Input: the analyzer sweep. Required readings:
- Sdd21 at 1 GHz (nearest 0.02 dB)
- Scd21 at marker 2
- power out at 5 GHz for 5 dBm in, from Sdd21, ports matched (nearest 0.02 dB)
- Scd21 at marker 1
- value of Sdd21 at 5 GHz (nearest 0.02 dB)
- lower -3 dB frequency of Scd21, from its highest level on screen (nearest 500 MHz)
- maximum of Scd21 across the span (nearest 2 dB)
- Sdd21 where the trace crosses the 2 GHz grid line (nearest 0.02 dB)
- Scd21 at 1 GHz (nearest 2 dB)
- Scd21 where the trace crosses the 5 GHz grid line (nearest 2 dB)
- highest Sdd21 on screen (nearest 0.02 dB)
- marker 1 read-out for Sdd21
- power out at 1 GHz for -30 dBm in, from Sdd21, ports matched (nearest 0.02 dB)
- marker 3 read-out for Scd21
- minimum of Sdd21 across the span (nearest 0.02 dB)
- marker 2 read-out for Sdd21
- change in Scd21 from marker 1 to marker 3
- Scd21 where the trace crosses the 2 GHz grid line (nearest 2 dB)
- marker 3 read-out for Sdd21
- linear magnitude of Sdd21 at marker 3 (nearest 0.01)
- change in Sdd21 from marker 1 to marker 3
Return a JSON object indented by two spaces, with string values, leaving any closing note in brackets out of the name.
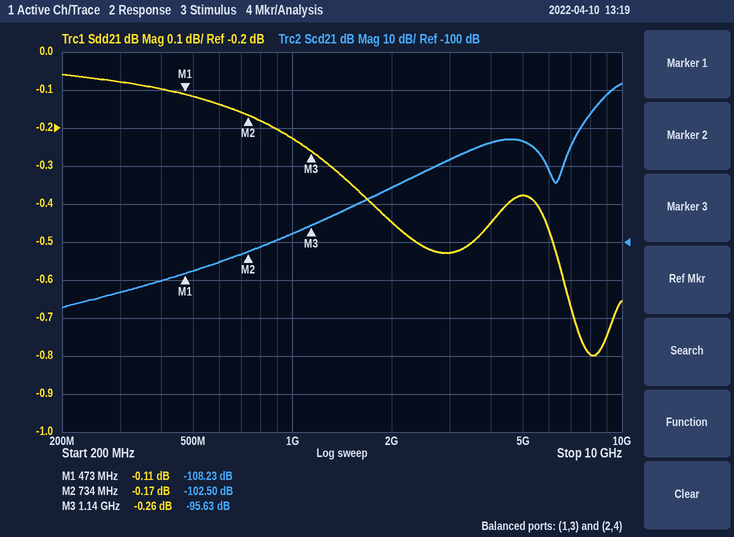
{
  "Sdd21 at 1 GHz": "-0.22 dB",
  "Scd21 at marker 2": "-102.50 dB",
  "power out at 5 GHz for 5 dBm in, from Sdd21, ports matched": "4.62 dBm",
  "Scd21 at marker 1": "-108.23 dB",
  "value of Sdd21 at 5 GHz": "-0.38 dB",
  "lower -3 dB frequency of Scd21, from its highest level on screen": "9.0 GHz",
  "maximum of Scd21 across the span": "-58 dB",
  "Sdd21 where the trace crosses the 2 GHz grid line": "-0.44 dB",
  "Scd21 at 1 GHz": "-98 dB",
  "Scd21 where the trace crosses the 5 GHz grid line": "-74 dB",
  "highest Sdd21 on screen": "-0.06 dB",
  "marker 1 read-out for Sdd21": "-0.11 dB",
  "power out at 1 GHz for -30 dBm in, from Sdd21, ports matched": "-30.22 dBm",
  "marker 3 read-out for Scd21": "-95.63 dB",
  "minimum of Sdd21 across the span": "-0.80 dB",
  "marker 2 read-out for Sdd21": "-0.17 dB",
  "change in Scd21 from marker 1 to marker 3": "12.60 dB",
  "Scd21 where the trace crosses the 2 GHz grid line": "-86 dB",
  "marker 3 read-out for Sdd21": "-0.26 dB",
  "linear magnitude of Sdd21 at marker 3": "0.97",
  "change in Sdd21 from marker 1 to marker 3": "-0.15 dB"
}
